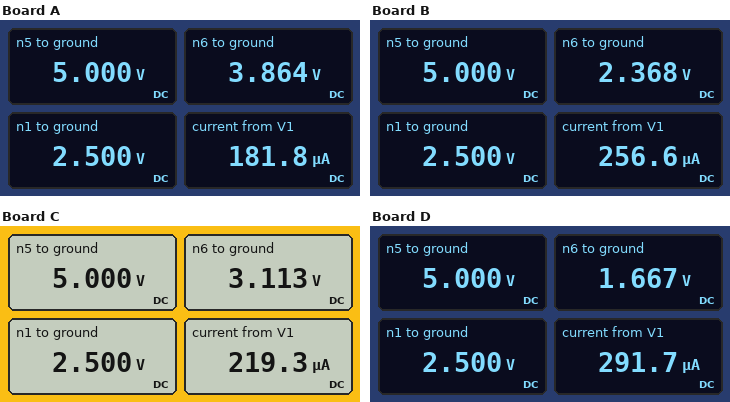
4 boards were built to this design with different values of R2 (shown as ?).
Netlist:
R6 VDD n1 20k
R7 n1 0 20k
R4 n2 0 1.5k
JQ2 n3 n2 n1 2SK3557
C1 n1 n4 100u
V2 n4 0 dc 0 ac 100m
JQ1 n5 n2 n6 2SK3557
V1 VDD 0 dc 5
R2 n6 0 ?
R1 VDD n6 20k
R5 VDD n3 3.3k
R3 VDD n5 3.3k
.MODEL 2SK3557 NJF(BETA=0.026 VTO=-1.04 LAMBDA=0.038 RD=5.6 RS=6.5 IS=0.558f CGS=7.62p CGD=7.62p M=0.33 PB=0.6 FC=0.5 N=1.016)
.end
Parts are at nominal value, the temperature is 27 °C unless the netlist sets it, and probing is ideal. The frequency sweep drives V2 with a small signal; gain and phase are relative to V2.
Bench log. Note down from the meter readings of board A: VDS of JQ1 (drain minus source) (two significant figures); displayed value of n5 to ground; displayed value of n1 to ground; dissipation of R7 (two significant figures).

1.1 V
5.000 V
2.500 V
310 µW
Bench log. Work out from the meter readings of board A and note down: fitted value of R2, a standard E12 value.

68 kΩ
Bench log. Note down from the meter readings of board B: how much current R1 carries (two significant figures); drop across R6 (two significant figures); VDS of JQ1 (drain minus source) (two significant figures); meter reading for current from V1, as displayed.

130 µA
2.5 V
2.6 V
256.6 µA
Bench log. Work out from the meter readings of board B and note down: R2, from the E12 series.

18 kΩ
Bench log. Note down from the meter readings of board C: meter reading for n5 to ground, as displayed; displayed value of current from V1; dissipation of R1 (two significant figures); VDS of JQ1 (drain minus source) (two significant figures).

5.000 V
219.3 µA
180 µW
1.9 V
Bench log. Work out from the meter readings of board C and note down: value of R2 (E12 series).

33 kΩ
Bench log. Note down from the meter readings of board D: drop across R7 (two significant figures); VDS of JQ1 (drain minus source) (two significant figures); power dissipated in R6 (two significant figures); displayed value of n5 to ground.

2.5 V
3.3 V
310 µW
5.000 V
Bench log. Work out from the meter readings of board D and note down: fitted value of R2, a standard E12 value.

10 kΩ
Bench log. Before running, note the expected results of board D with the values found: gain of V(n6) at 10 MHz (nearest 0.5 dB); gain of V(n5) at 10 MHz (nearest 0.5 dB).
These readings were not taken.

-15.5 dB
-20.5 dB
